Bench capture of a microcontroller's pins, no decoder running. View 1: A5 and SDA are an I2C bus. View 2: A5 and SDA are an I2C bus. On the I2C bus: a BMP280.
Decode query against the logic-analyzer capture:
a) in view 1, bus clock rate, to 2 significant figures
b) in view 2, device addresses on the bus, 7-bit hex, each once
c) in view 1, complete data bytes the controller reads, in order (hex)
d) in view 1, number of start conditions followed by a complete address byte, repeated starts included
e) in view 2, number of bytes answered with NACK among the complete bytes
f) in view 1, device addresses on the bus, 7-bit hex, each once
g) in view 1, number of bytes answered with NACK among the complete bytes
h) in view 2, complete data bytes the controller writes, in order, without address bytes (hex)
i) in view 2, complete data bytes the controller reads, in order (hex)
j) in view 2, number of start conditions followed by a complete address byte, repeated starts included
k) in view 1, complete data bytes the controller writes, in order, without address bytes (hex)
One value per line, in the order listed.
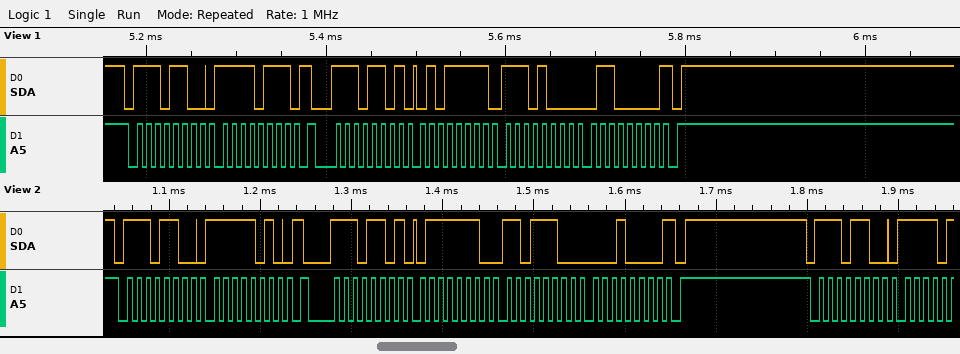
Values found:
100 kHz
0x76
5F E8 60
2
1
0x76
1
FA
7E DC 10
3
F7
